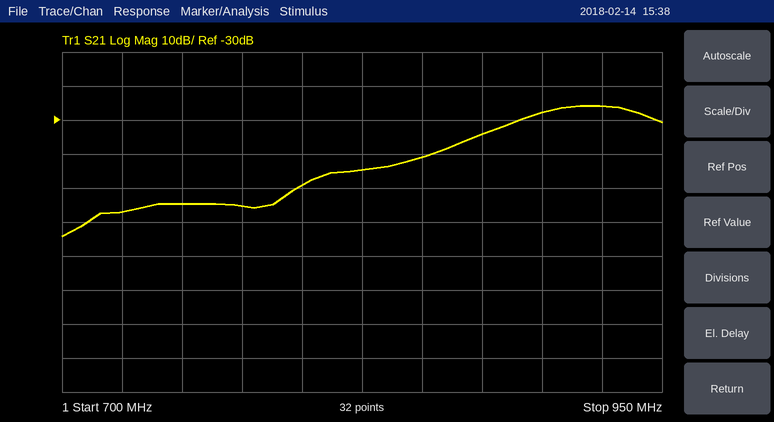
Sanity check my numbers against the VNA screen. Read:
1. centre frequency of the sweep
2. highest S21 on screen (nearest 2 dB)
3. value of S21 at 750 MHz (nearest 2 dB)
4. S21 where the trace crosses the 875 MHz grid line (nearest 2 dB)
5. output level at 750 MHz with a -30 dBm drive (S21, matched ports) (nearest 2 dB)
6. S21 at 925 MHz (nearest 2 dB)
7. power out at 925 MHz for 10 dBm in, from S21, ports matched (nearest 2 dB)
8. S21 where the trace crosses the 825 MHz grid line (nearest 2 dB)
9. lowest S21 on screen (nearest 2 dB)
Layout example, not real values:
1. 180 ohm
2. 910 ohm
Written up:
1. 825 MHz
2. -26 dB
3. -54 dB
4. -34 dB
5. -84 dBm
6. -26 dB
7. -16 dBm
8. -44 dB
9. -64 dB
